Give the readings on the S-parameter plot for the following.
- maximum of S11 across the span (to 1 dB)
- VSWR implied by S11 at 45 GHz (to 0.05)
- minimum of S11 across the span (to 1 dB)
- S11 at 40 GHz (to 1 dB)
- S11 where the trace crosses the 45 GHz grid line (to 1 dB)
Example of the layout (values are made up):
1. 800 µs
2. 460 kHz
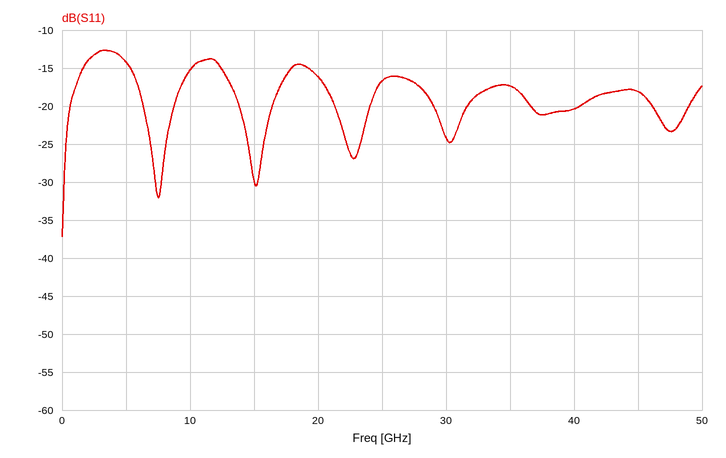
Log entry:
1. -13 dB
2. 1.30
3. -37 dB
4. -20 dB
5. -18 dB
